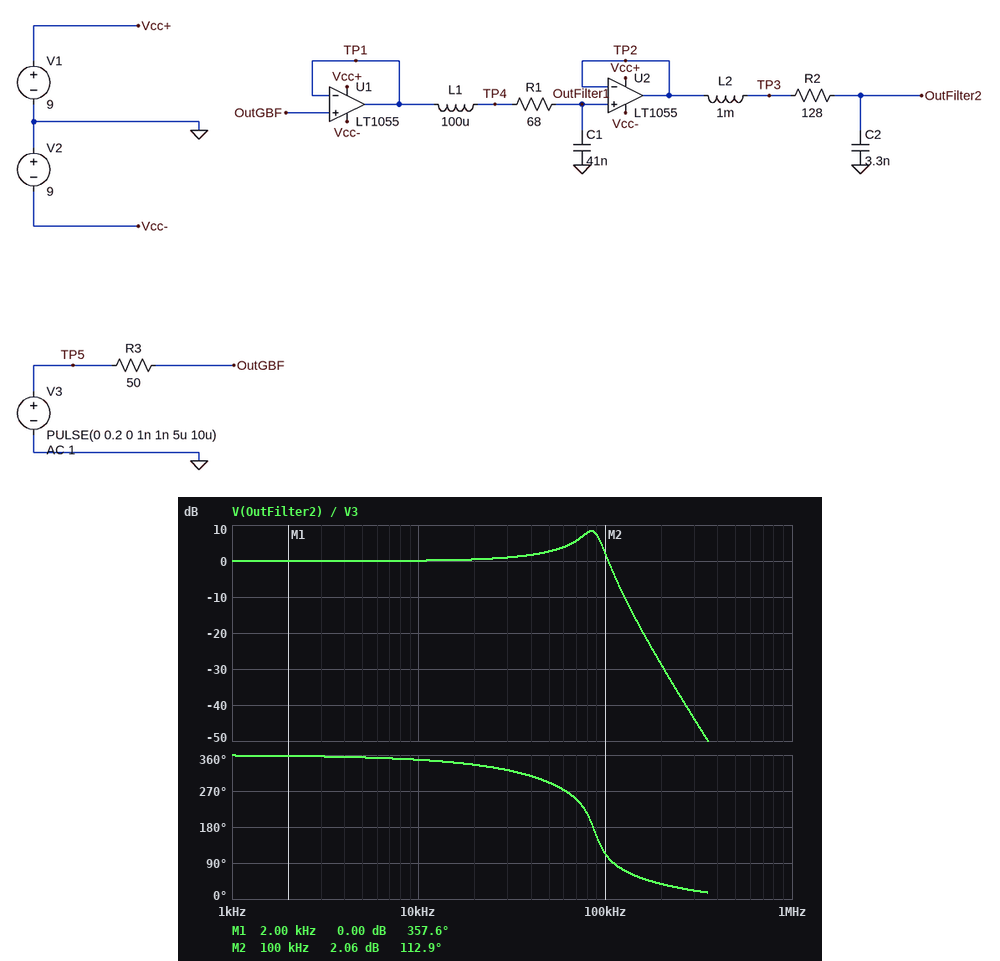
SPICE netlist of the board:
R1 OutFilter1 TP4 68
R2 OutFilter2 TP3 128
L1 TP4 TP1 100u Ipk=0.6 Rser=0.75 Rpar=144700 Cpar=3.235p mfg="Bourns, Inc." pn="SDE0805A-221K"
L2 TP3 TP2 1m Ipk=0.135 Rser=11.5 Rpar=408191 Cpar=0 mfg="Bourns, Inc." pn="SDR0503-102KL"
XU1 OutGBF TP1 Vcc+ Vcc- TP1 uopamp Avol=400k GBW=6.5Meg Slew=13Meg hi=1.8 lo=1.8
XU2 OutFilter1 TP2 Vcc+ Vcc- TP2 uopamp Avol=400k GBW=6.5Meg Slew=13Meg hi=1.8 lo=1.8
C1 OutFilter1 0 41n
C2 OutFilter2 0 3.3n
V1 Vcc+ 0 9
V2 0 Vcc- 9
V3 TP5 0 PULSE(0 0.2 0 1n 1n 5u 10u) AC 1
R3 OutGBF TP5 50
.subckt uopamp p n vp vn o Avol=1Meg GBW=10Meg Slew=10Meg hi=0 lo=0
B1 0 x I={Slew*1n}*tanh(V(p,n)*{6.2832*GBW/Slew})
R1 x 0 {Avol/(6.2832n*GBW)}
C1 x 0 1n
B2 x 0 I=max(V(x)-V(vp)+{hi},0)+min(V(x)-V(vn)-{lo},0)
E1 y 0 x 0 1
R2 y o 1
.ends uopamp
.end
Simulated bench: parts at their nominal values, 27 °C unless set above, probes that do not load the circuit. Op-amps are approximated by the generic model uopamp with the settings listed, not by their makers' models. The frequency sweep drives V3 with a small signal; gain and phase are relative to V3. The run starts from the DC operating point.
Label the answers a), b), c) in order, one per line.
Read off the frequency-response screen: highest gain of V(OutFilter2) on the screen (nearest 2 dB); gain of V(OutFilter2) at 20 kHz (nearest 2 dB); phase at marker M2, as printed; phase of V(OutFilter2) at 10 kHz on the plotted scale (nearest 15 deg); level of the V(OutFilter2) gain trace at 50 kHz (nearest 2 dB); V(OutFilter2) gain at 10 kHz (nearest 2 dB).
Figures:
a) 8 dB
b) 0 dB
c) 112.9 deg
d) 345 deg
e) 2 dB
f) 0 dB
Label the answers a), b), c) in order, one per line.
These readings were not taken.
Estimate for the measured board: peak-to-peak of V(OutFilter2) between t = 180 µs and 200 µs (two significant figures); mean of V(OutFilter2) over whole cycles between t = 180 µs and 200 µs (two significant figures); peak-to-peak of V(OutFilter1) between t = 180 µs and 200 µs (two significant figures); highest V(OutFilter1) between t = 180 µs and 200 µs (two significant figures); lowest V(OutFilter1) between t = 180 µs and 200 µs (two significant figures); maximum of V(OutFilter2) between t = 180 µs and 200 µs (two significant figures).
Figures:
a) 320 mV
b) 100 mV
c) 140 mV
d) 170 mV
e) 29 mV
f) 260 mV
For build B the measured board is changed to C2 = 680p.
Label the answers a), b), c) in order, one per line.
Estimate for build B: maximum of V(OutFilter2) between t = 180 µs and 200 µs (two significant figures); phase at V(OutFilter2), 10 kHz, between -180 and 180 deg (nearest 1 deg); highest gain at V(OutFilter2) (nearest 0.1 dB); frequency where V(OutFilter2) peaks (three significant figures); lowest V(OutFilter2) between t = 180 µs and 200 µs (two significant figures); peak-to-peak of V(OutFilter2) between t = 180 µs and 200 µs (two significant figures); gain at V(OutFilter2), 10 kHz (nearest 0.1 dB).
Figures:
a) 190 mV
b) -11 deg
c) 3.0 dB
d) 191 kHz
e) 9.6 mV
f) 180 mV
g) 0 dB
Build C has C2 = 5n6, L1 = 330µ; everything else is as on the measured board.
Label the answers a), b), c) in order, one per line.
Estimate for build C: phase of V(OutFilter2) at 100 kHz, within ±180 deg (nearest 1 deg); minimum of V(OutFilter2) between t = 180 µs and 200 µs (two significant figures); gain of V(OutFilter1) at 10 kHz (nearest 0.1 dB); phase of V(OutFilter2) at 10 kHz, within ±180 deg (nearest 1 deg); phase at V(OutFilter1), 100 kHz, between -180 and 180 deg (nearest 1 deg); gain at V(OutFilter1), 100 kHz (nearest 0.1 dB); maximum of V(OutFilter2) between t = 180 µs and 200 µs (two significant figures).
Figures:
a) 43 deg
b) 79 mV
c) 0.3 dB
d) -14 deg
e) -159 deg
f) -13.4 dB
g) 120 mV
